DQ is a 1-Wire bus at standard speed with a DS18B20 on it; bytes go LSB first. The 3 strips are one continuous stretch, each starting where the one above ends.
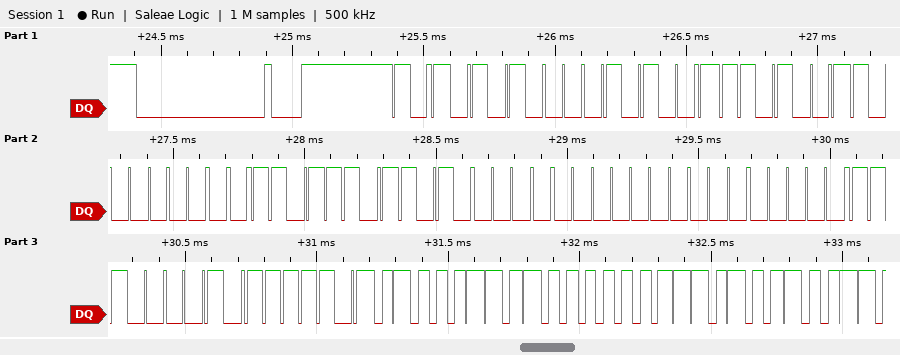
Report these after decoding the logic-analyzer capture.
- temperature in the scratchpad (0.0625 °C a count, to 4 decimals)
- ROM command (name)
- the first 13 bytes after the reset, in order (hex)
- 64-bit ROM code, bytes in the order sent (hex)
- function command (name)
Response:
22.1250 °C
Match ROM
55 28 97 01 76 0B 00 00 87 BE 62 01 4B
28 97 01 76 0B 00 00 87
Read Scratchpad
